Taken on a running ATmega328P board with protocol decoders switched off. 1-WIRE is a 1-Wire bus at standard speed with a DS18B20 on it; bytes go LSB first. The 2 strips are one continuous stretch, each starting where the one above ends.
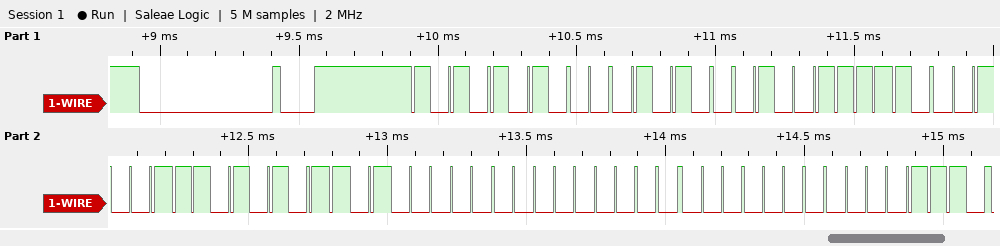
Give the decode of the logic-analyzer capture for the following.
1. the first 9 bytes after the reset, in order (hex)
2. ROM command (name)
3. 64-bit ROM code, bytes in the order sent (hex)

55 28 F2 91 AB 05 00 00 70
Match ROM
28 F2 91 AB 05 00 00 70
